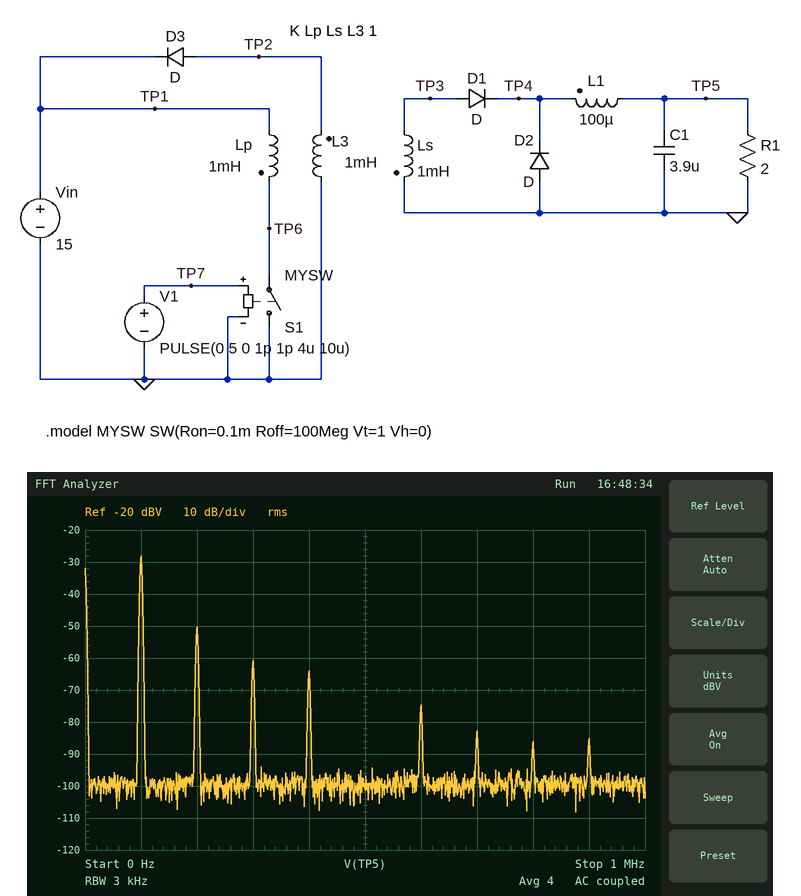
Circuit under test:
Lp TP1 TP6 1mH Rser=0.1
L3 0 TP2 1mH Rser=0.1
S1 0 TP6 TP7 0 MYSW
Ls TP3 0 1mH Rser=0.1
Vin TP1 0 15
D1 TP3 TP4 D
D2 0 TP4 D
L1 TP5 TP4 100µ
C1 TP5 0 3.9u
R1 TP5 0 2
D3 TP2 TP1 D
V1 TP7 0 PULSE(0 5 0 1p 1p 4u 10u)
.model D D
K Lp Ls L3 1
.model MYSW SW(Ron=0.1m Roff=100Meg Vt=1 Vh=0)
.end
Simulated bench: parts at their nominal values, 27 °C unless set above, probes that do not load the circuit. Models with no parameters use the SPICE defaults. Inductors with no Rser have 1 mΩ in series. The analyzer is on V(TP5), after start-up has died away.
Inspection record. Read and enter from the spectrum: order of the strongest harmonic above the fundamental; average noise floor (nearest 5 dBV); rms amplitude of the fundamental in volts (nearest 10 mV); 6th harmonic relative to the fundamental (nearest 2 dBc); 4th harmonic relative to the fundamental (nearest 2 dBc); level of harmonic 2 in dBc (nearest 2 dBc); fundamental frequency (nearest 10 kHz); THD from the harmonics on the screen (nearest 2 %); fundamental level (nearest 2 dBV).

2
-100 dBV
40 mV
-46 dBc
-36 dBc
-22 dBc
100 kHz
8 %
-28 dBV
